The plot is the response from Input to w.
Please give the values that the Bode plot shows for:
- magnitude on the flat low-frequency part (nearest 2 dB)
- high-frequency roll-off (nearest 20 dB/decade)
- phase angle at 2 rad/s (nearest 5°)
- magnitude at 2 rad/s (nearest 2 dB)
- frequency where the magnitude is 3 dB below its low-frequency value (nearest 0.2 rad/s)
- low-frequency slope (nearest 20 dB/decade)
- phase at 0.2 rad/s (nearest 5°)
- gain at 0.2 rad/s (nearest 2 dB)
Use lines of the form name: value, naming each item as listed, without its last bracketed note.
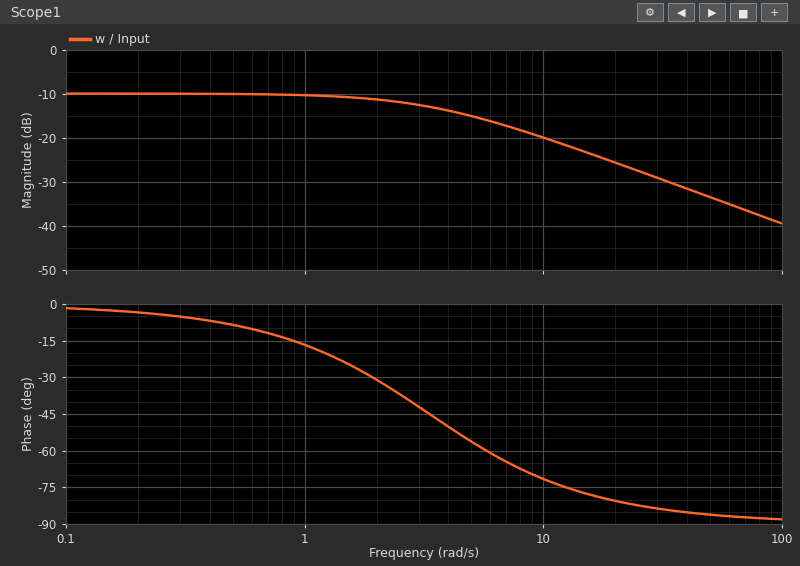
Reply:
magnitude on the flat low-frequency part: -10 dB
high-frequency roll-off: -20 dB/decade
phase angle at 2 rad/s: -30°
magnitude at 2 rad/s: -12 dB
frequency where the magnitude is 3 dB below its low-frequency value: 3.4 rad/s
low-frequency slope: 0 dB/decade
phase at 0.2 rad/s: -5°
gain at 0.2 rad/s: -10 dB
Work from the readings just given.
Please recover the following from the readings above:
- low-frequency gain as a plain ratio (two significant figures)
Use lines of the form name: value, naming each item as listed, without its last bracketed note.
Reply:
low-frequency gain as a plain ratio: 0.32
